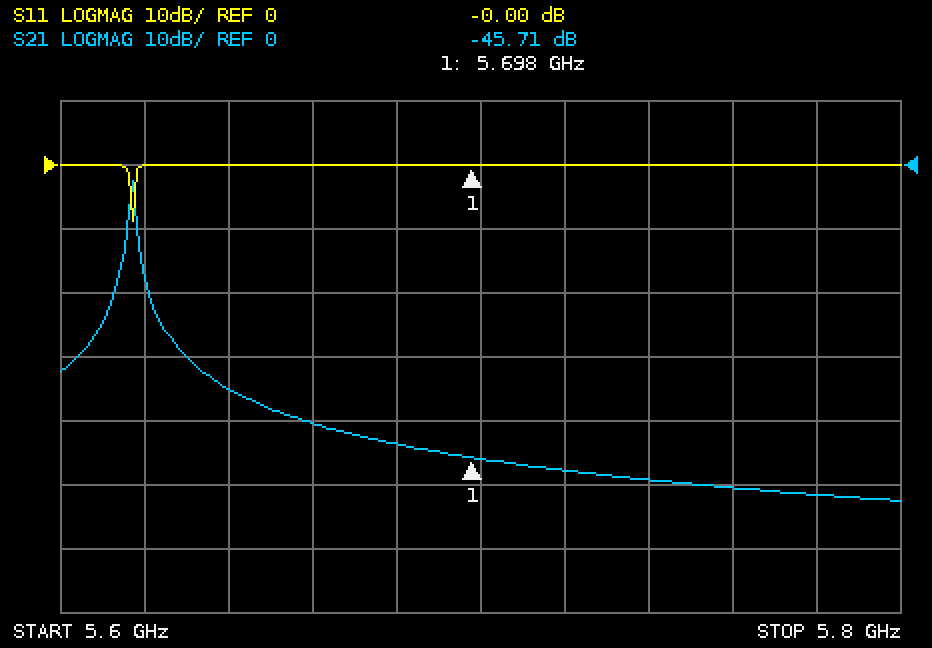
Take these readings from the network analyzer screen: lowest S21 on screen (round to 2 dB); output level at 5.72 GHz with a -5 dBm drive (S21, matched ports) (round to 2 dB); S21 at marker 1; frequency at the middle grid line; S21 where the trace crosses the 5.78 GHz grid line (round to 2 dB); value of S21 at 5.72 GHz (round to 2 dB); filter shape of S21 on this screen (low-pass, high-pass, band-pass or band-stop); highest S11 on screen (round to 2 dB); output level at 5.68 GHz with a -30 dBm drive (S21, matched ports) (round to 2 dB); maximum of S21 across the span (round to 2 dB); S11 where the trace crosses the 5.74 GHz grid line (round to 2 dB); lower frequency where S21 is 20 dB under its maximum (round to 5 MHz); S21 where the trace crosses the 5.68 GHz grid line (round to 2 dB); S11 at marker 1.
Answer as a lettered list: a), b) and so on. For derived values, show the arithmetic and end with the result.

a) -52 dB
b) -5 dBm + (-48 dB) = -52 dBm
c) -45.71 dB
d) 5.7 GHz
e) -52 dB
f) -48 dB
g) band-pass
h) 0 dB
i) -30 dBm + (-44 dB) = -74 dBm
j) -2 dB
k) 0 dB
l) 5.610 GHz
m) -44 dB
n) -0.00 dB
